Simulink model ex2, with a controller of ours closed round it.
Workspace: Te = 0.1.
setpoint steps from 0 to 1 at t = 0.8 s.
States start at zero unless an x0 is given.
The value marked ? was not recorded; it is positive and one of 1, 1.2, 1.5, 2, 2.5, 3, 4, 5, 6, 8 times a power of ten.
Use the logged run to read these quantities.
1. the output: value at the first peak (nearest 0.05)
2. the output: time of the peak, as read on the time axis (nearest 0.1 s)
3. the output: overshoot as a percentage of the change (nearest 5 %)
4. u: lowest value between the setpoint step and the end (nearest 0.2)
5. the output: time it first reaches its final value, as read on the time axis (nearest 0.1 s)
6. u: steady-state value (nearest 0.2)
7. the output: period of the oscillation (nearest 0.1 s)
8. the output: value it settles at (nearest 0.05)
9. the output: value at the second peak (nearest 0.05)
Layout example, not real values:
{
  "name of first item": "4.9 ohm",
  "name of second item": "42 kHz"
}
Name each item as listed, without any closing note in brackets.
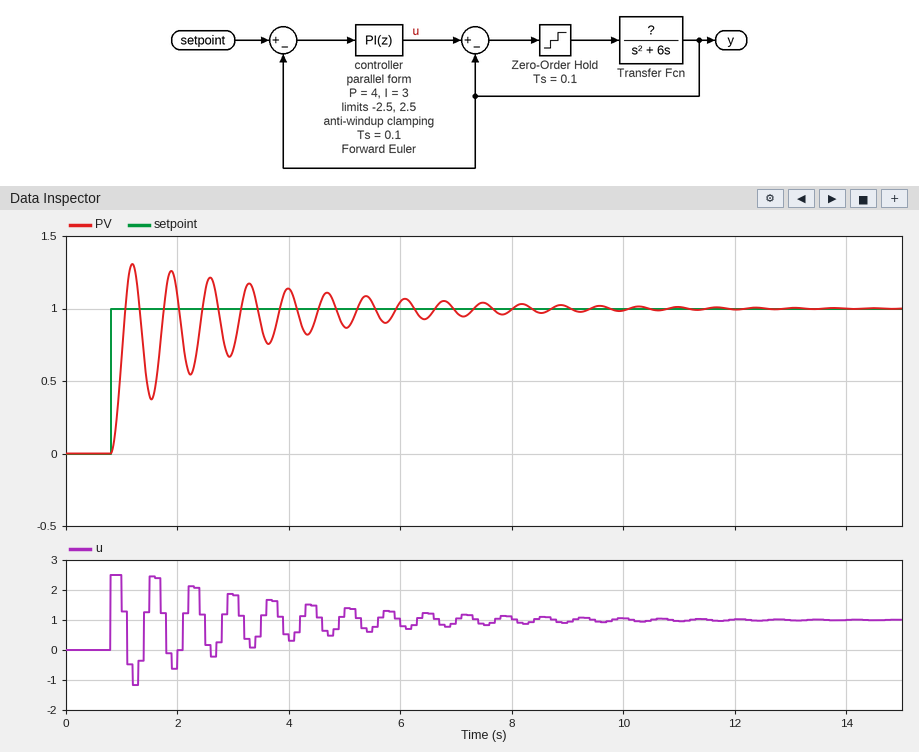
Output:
{
  "the output: value at the first peak": "1.30",
  "the output: time of the peak, as read on the time axis": "1.2 s",
  "the output: overshoot as a percentage of the change": "30 %",
  "u: lowest value between the setpoint step and the end": "-1.2",
  "the output: time it first reaches its final value, as read on the time axis": "1.1 s",
  "u: steady-state value": "1.0",
  "the output: period of the oscillation": "0.7 s",
  "the output: value it settles at": "1.00",
  "the output: value at the second peak": "1.25"
}
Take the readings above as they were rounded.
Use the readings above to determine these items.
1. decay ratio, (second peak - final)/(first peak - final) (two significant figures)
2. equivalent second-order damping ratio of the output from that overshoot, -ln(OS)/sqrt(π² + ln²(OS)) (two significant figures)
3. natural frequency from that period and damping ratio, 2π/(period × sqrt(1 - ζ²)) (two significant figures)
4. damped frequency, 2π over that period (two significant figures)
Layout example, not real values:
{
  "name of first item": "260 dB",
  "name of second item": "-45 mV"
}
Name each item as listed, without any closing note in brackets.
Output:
{
  "decay ratio, (second peak - final)/(first peak - final)": "0.83",
  "equivalent second-order damping ratio of the output from that overshoot, -ln(OS)/sqrt(π² + ln²(OS))": "0.36",
  "natural frequency from that period and damping ratio, 2π/(period × sqrt(1 - ζ²))": "9.6 rad/s",
  "damped frequency, 2π over that period": "9.0 rad/s"
}
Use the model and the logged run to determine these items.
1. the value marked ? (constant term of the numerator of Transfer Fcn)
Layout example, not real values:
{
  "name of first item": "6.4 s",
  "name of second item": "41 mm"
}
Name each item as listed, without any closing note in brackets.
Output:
{
  "the value marked ?": "20"
}
